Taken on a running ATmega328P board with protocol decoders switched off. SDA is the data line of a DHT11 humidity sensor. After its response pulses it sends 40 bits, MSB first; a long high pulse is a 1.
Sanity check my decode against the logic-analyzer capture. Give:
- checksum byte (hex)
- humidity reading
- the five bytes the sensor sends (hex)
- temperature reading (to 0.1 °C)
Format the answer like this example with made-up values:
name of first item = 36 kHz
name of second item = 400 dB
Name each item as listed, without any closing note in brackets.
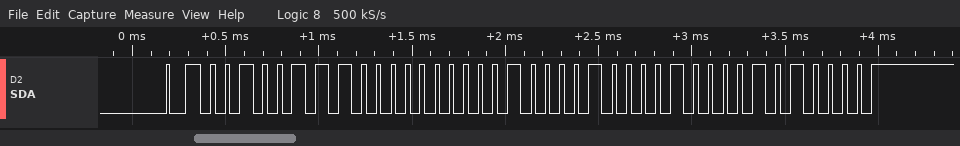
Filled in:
checksum byte = 0x50
humidity reading = 39 %
the five bytes the sensor sends = 27 00 21 08 50
temperature reading = 33.8 °C
